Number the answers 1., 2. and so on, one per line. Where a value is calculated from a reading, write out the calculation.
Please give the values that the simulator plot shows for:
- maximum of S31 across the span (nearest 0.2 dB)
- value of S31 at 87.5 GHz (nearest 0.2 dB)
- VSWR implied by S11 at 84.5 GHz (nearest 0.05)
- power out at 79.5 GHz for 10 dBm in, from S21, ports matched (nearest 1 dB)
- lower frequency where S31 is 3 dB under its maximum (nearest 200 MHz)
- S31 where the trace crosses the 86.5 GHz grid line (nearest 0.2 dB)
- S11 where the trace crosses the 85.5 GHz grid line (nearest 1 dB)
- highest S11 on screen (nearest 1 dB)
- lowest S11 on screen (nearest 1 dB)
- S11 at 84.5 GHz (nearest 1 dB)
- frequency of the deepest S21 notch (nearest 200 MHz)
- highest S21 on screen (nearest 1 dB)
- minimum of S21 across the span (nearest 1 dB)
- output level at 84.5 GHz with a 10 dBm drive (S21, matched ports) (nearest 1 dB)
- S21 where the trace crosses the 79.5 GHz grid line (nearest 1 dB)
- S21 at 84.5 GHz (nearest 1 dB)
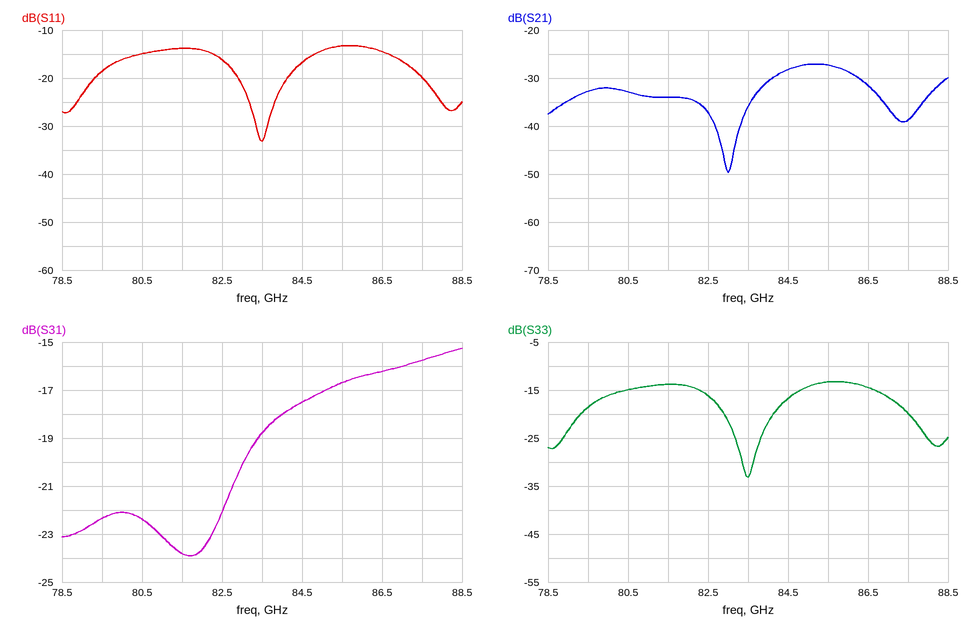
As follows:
1. -15.2 dB
2. -15.8 dB
3. |Γ| = 10^(-17/20) = 0.1413; VSWR = (1 + 0.1413)/(1 − 0.1413) ≈ 1.33, so 1.35 to the nearest 0.05
4. 10 dBm + (-33 dB) = -23 dBm
5. 83.8 GHz
6. -16.2 dB
7. -13 dB
8. -13 dB
9. -33 dB
10. -17 dB
11. 83.0 GHz
12. -27 dB
13. -50 dB
14. 10 dBm + (-28 dB) = -18 dBm
15. -33 dB
16. -28 dB
